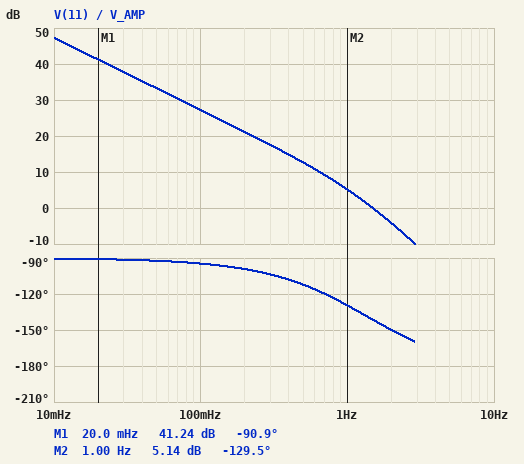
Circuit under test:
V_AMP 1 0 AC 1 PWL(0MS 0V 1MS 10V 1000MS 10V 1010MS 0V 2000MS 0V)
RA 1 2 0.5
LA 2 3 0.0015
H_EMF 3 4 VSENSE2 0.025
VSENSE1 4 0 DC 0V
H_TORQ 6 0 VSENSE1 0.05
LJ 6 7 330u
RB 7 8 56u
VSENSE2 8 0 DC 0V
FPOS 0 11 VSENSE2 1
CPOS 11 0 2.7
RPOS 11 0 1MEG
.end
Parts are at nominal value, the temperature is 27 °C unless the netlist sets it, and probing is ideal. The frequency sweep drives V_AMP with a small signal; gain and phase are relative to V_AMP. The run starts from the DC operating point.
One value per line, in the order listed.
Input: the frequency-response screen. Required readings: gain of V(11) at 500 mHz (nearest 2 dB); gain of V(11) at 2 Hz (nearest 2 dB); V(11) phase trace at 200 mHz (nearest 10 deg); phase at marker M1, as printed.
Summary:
12 dB
-4 dB
-100 deg
-90.9 deg
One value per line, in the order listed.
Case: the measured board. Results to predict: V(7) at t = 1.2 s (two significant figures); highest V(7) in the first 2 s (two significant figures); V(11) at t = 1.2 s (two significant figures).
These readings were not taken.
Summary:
4.8 mV
22 mV
140 V
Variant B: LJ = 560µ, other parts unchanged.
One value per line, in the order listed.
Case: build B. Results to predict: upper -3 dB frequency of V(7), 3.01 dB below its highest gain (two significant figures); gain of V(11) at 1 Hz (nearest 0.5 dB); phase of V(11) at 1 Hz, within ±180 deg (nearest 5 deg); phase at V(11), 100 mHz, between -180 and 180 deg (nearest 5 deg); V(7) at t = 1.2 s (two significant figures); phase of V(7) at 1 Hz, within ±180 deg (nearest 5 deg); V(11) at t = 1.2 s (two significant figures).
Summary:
740 mHz
2.5 dB
-145 deg
-100 deg
8.9 mV
-55 deg
130 V
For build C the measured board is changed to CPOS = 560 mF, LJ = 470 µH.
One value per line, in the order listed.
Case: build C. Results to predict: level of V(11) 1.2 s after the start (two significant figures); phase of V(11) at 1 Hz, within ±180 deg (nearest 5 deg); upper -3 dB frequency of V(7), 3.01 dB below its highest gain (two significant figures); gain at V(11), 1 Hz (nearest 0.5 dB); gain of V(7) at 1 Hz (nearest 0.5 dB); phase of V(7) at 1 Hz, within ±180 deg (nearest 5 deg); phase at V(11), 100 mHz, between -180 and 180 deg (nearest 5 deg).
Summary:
660 V
-140 deg
880 mHz
17.5 dB
-57.0 dB
-50 deg
-95 deg
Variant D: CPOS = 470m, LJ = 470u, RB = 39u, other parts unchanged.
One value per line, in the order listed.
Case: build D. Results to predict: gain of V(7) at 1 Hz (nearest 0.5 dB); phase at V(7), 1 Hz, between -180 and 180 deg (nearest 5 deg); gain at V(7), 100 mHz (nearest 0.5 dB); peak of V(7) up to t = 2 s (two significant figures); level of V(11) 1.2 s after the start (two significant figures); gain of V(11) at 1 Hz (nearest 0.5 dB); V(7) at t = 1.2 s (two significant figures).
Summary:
-60.0 dB
-50 deg
-56.5 dB
15 mV
790 V
19.0 dB
5.3 mV
